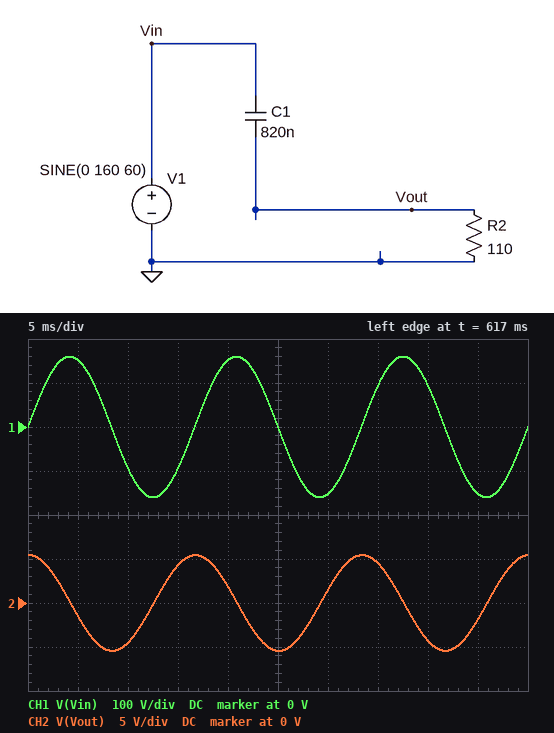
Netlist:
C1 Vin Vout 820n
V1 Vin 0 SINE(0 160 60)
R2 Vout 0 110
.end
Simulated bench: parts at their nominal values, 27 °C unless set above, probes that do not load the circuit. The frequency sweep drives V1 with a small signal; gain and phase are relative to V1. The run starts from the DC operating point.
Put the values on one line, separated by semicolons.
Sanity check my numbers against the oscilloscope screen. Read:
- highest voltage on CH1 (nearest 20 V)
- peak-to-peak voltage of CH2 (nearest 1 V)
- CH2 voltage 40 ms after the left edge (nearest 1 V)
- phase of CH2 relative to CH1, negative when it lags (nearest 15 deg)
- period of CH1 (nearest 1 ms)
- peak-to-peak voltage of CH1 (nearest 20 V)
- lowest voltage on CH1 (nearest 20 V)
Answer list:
160 V; 11 V; -4 V; 90 deg; 17 ms; 320 V; -160 V
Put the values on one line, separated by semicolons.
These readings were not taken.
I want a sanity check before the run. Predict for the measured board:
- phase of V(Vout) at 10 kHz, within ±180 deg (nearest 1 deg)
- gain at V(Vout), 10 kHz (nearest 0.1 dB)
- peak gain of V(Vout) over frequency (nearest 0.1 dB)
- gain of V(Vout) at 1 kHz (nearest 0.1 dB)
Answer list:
10 deg; -0.1 dB; 0 dB; -6.1 dB
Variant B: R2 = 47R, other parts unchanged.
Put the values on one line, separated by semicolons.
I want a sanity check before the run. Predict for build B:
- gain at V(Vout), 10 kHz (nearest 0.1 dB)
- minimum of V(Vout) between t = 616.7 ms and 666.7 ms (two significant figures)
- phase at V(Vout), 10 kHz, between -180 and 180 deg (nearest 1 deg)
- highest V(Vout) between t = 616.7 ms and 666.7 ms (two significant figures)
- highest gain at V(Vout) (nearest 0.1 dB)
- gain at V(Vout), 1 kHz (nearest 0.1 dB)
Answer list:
-0.7 dB; -2.3 V; 22 deg; 2.3 V; 0 dB; -12.6 dB
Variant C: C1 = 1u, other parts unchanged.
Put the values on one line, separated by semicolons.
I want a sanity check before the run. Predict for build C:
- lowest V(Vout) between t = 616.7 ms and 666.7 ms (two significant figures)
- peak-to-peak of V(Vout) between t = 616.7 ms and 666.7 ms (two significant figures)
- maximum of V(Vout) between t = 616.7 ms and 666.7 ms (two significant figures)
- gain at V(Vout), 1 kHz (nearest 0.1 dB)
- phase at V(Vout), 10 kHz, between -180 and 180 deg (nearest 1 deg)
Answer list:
-6.6 V; 13 V; 6.6 V; -4.9 dB; 8 deg
